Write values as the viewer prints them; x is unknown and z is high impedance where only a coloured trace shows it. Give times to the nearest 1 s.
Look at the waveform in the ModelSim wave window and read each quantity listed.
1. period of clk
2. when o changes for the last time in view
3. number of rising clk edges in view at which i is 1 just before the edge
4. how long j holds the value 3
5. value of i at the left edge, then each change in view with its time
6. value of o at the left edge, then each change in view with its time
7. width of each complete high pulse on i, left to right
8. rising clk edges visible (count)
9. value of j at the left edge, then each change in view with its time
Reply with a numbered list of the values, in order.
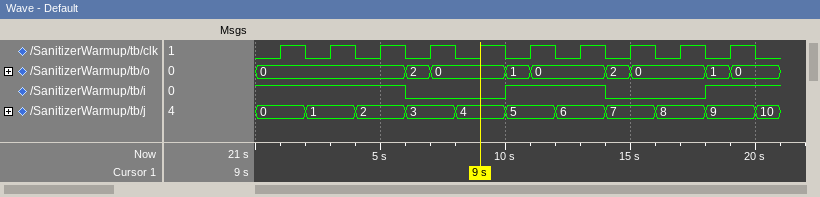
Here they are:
1. 2 s
2. 19 s
3. 6
4. 2 s
5. 1, 0 at 6 s, 1 at 10 s, 0 at 14 s, 1 at 18 s
6. 0, 2 at 6 s, 0 at 7 s, 1 at 10 s, 0 at 11 s, 2 at 14 s, 0 at 15 s, 1 at 18 s, 0 at 19 s
7. 4 s
8. 10
9. 0, 1 at 2 s, 2 at 4 s, 3 at 6 s, 4 at 8 s, 5 at 10 s, 6 at 12 s, 7 at 14 s, 8 at 16 s, 9 at 18 s, 10 at 20 s
